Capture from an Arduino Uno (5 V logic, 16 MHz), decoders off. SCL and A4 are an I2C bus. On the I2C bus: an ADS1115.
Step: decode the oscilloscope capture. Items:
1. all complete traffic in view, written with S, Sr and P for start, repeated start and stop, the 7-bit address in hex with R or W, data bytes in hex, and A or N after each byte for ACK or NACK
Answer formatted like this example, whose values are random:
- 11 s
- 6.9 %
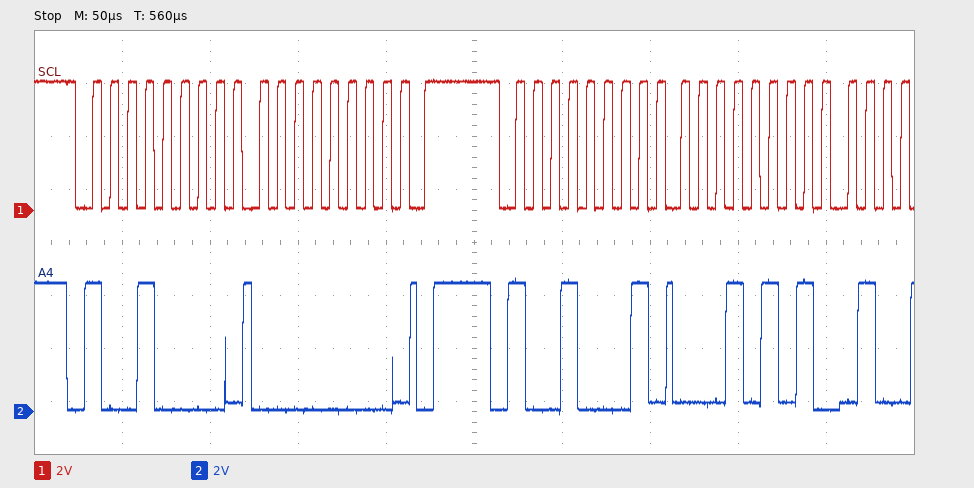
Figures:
- S 48W A 00 A P S 48R A 15 A
